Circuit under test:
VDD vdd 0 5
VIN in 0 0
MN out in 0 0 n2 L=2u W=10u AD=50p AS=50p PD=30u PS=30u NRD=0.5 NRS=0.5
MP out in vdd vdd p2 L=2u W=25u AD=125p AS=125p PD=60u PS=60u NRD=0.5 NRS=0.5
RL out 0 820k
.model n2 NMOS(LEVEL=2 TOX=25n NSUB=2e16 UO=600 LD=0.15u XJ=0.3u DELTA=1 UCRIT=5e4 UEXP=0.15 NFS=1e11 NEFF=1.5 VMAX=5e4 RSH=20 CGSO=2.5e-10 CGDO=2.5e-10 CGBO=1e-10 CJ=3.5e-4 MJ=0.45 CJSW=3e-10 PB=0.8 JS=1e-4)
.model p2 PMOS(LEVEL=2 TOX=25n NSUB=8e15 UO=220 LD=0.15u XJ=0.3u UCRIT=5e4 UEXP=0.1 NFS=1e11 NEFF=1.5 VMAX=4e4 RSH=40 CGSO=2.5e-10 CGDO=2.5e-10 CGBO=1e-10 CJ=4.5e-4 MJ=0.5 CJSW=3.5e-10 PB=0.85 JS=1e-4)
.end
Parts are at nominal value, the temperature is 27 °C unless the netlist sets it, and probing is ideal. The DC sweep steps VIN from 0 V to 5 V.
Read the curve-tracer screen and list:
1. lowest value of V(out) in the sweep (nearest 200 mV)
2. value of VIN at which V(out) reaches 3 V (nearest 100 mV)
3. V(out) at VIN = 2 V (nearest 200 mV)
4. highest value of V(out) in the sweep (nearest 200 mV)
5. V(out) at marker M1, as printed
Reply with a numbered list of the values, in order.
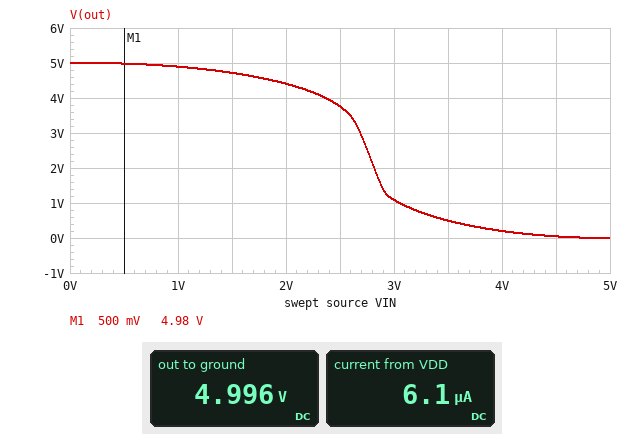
1. 0 V
2. 2.7 V
3. 4.4 V
4. 5.0 V
5. 4.98 V
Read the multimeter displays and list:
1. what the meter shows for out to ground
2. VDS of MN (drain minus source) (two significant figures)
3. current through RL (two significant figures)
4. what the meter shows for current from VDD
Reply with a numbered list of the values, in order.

1. 4.996 V
2. 5.0 V
3. 6.1 µA
4. 6.1 µA
